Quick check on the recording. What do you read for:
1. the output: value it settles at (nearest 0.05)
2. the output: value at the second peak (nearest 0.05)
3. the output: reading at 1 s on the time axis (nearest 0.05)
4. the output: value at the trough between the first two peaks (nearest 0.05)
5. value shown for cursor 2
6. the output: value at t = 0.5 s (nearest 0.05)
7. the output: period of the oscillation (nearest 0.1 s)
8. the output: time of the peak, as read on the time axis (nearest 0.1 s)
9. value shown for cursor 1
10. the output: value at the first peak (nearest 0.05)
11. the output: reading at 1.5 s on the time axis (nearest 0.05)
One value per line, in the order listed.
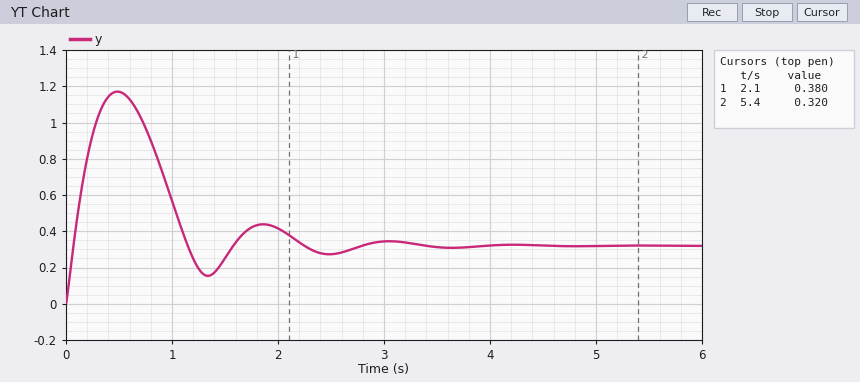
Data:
0.30
0.45
0.55
0.15
0.320
1.15
1.4 s
0.5 s
0.380
1.15
0.25
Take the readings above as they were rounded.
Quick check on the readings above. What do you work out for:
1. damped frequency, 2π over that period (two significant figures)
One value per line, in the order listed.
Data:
4.5 rad/s
